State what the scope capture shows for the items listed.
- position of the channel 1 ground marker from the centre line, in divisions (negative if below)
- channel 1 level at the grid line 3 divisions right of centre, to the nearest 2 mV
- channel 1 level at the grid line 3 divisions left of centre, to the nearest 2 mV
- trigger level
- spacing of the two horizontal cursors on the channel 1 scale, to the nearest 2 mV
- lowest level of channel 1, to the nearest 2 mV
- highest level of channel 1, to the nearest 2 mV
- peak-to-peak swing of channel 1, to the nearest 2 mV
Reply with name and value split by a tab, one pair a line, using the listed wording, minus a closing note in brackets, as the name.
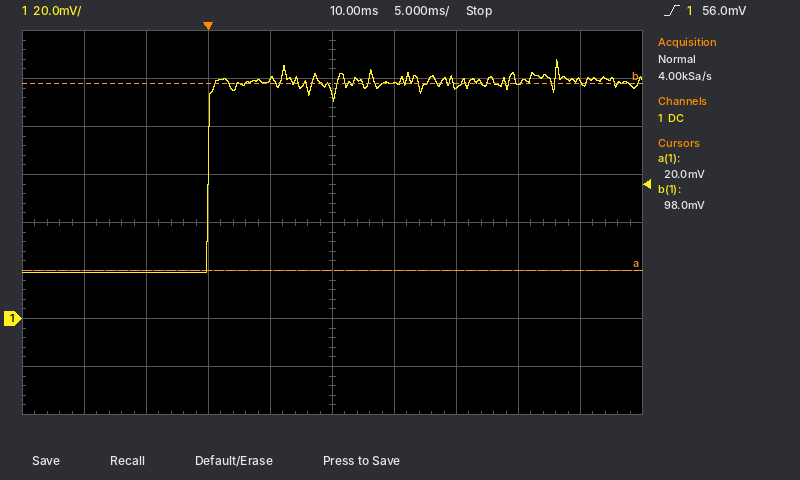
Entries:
position of the channel 1 ground marker from the centre line, in divisions	-2.0 div
channel 1 level at the grid line 3 divisions right of centre, to the nearest 2 mV	98 mV
channel 1 level at the grid line 3 divisions left of centre, to the nearest 2 mV	20 mV
trigger level	56.0 mV
spacing of the two horizontal cursors on the channel 1 scale, to the nearest 2 mV	78 mV
lowest level of channel 1, to the nearest 2 mV	20 mV
highest level of channel 1, to the nearest 2 mV	108 mV
peak-to-peak swing of channel 1, to the nearest 2 mV	88 mV
